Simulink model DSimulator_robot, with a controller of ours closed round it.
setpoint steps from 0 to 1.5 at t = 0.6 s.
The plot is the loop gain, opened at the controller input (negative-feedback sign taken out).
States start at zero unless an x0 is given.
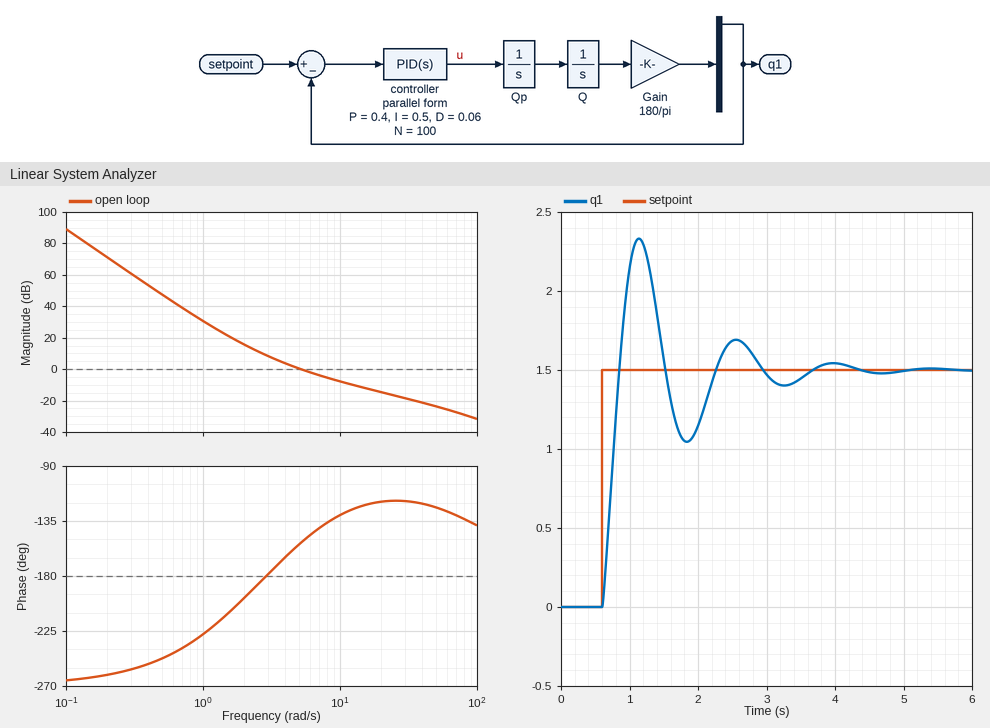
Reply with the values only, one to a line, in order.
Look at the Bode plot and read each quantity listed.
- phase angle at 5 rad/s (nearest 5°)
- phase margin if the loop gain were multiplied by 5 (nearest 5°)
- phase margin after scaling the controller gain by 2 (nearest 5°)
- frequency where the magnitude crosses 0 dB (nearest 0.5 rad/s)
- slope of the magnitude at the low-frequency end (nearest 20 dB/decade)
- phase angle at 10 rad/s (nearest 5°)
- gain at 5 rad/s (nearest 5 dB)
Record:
-155°
60°
45°
5.0 rad/s
-60 dB/decade
-130°
0 dB
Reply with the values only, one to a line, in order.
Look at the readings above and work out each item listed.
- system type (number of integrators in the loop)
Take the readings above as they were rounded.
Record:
3
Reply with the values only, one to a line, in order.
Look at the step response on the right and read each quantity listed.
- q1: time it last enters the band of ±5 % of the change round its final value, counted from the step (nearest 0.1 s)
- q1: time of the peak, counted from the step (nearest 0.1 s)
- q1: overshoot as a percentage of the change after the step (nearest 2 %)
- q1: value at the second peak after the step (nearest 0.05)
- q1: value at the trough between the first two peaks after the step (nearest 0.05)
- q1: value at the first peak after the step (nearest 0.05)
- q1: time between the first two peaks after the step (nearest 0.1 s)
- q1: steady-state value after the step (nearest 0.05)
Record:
2.8 s
0.5 s
56 %
1.70
1.05
2.35
1.4 s
1.50
